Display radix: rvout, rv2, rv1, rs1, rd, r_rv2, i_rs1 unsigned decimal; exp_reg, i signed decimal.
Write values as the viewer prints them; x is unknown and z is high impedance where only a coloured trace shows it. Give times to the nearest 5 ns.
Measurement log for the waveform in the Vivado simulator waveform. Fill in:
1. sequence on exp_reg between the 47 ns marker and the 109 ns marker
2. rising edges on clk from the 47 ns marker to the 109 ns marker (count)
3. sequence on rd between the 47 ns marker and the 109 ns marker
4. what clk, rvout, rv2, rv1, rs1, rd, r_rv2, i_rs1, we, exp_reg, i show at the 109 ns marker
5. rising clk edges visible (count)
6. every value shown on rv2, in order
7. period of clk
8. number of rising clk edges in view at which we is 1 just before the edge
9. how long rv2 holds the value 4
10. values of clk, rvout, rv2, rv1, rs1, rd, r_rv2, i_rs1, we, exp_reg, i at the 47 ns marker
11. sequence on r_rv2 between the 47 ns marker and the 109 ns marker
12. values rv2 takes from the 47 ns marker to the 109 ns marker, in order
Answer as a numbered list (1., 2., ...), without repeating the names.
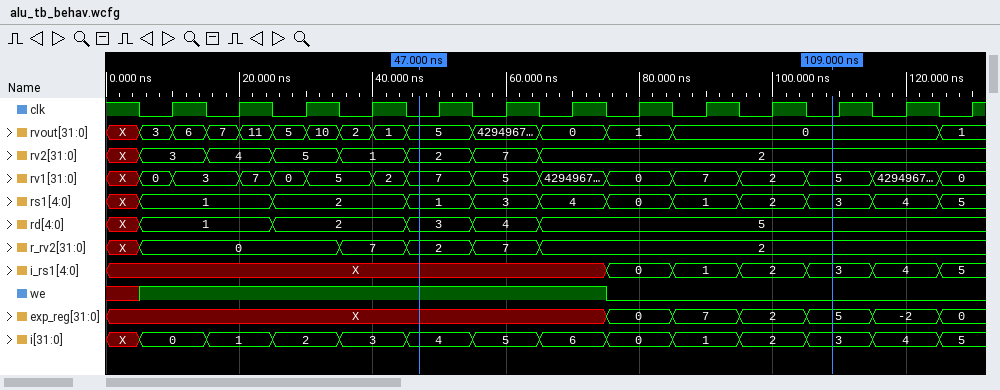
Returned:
1. X, 0, 7, 2, 5
2. 6
3. 3, 4, 5
4. clk=0, rvout=0, rv2=2, rv1=5, rs1=3, rd=5, r_rv2=2, i_rs1=3, we=0, exp_reg=5, i=3
5. 13
6. X, 3, 4, 5, 1, 2, 7, 2
7. 10 ns
8. 7
9. 10 ns
10. clk=0, rvout=5, rv2=2, rv1=7, rs1=1, rd=3, r_rv2=2, i_rs1=X, we=1, exp_reg=X, i=4
11. 2, 7, 2
12. 2, 7, 2
